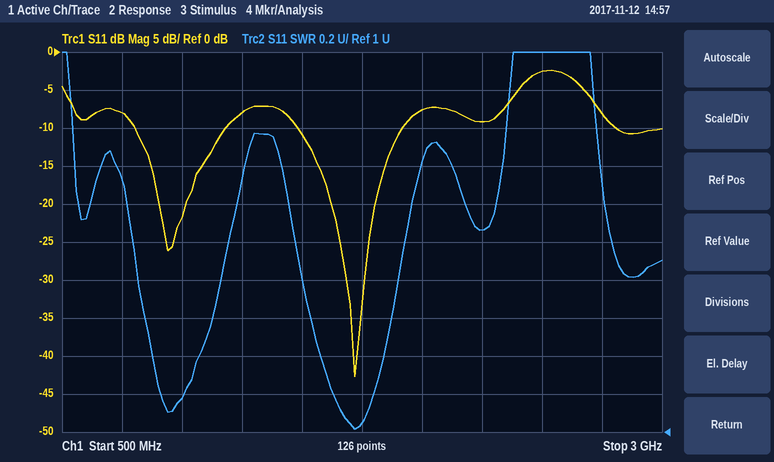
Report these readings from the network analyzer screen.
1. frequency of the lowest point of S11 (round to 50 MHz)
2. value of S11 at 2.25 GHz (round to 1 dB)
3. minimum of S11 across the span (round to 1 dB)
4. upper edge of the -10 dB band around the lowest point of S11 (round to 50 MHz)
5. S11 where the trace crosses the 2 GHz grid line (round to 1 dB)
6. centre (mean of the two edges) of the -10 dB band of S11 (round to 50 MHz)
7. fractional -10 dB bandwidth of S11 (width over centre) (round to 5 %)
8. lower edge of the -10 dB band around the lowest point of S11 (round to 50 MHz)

1.70 GHz
-9 dB
-43 dB
1.90 GHz
-8 dB
1.70 GHz
25 %
1.50 GHz
